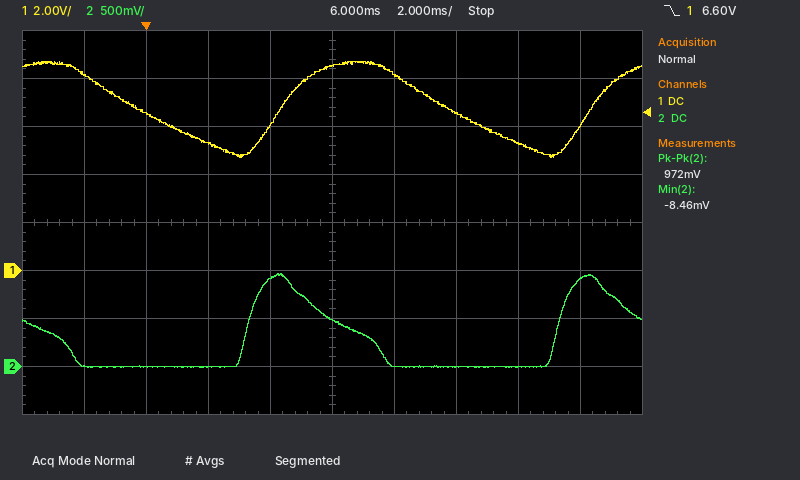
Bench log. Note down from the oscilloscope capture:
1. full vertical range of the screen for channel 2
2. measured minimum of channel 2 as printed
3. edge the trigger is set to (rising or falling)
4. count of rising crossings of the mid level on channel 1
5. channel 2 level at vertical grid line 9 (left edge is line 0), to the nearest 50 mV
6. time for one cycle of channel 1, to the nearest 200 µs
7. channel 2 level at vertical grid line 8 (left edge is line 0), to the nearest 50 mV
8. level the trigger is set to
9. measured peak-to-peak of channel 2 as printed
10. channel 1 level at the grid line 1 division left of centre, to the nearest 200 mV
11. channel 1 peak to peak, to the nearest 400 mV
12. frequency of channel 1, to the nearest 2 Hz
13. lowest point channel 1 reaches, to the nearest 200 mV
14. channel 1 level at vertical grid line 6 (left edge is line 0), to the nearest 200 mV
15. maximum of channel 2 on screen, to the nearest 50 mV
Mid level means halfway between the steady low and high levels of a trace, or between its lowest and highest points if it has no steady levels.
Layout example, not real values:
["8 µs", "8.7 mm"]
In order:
["4 V", "-8.46 mV", "falling", "2", "900 mV", "10.0 ms", "0 mV", "6.60 V", "972 mV", "6.0 V", "4.0 V", "100 Hz", "4.8 V", "8.2 V", "950 mV"]
